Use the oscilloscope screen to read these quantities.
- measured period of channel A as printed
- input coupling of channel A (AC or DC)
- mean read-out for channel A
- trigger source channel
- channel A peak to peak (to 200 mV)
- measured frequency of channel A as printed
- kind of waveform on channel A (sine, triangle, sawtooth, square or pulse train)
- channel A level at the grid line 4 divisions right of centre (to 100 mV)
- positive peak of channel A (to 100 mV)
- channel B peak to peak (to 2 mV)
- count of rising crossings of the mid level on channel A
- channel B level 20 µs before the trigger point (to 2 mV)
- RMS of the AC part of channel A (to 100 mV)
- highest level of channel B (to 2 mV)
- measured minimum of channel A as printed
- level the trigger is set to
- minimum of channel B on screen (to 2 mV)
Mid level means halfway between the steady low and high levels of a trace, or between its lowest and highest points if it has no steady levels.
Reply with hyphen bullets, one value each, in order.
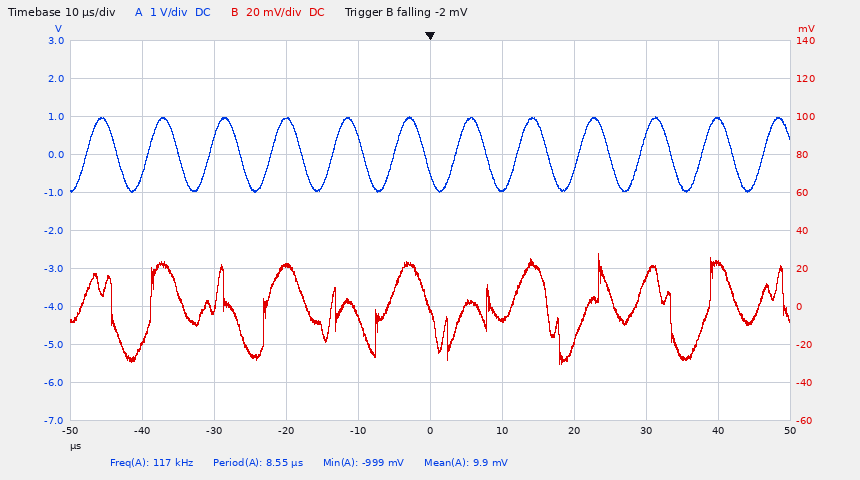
- 8.55 µs
- DC
- 9.9 mV
- channel B
- 2.0 V
- 117 kHz
- sine
- 900 mV
- 1.0 V
- 58 mV
- 12
- 22 mV
- 700 mV
- 28 mV
- -999 mV
- -2 mV
- -30 mV
